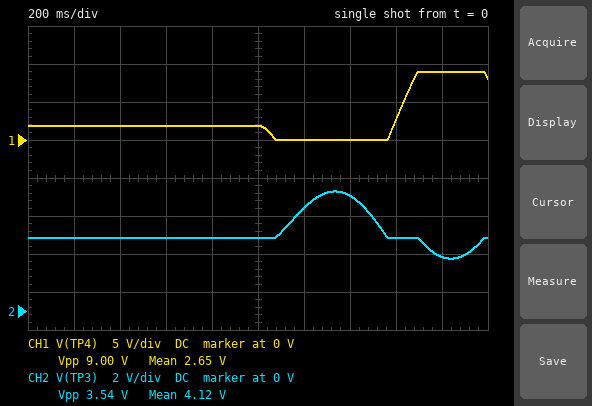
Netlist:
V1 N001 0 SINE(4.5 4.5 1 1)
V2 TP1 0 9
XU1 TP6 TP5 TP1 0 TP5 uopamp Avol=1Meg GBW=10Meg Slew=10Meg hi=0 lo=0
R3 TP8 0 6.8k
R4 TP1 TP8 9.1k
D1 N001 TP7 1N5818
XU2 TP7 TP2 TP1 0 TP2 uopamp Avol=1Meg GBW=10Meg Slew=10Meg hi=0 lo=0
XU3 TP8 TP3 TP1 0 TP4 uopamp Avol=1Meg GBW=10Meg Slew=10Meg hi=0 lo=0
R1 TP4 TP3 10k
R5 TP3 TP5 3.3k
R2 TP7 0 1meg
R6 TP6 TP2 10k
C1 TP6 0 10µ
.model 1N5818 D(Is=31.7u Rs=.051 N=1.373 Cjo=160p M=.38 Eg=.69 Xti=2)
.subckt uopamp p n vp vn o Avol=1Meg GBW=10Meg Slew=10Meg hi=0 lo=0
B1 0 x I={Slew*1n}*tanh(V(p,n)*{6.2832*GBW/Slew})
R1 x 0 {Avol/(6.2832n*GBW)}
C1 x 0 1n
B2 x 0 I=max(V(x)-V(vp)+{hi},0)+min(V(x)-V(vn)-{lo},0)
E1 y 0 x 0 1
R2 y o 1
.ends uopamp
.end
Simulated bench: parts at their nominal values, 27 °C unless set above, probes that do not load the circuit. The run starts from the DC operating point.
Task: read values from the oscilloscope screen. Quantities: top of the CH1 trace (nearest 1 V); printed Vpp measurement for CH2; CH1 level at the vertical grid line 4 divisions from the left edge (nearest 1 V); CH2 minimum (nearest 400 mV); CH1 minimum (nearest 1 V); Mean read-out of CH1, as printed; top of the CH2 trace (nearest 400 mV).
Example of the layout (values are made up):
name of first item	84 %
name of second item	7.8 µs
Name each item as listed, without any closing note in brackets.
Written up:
top of the CH1 trace	9 V
printed Vpp measurement for CH2	3.54 V
CH1 level at the vertical grid line 4 divisions from the left edge	2 V
CH2 minimum	2.8 V
CH1 minimum	0 V
Mean read-out of CH1, as printed	2.65 V
top of the CH2 trace	6.4 V
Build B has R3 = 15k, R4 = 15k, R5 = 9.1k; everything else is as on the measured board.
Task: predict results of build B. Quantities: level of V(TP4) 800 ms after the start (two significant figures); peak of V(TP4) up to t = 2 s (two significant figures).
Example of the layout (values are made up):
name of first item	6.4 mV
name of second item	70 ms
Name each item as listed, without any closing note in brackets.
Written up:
level of V(TP4) 800 ms after the start	4.5 V
peak of V(TP4) up to t = 2 s	8.7 V
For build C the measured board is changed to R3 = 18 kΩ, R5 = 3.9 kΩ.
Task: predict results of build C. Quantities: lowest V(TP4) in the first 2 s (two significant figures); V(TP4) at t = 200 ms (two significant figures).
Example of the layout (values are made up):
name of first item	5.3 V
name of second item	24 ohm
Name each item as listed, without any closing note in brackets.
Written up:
lowest V(TP4) in the first 2 s	-2.1 mV
V(TP4) at t = 200 ms	9.0 V
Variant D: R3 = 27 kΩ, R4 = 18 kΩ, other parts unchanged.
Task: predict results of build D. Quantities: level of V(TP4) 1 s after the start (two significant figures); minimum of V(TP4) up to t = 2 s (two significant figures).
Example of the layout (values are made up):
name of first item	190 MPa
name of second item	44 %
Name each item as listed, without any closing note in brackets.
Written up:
level of V(TP4) 1 s after the start	8.1 V
minimum of V(TP4) up to t = 2 s	-9.4 mV
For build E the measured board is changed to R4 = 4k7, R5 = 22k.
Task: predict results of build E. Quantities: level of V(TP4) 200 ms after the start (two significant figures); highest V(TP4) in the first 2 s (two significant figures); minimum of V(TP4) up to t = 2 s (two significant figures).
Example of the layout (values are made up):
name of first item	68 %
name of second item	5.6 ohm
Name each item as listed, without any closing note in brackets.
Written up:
level of V(TP4) 200 ms after the start	5.7 V
highest V(TP4) in the first 2 s	7.4 V
minimum of V(TP4) up to t = 2 s	3.9 V
